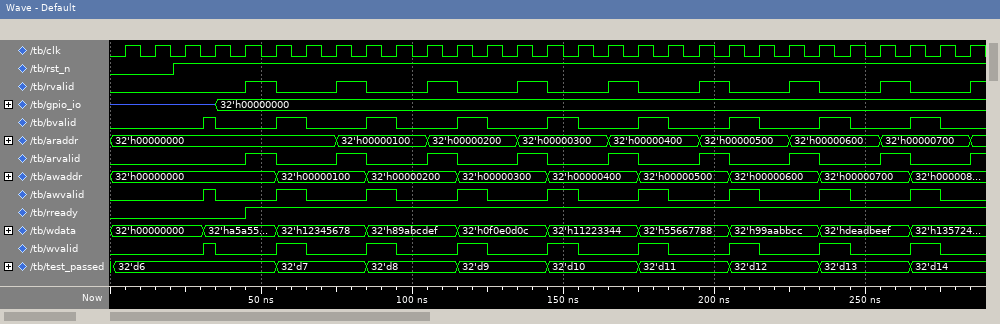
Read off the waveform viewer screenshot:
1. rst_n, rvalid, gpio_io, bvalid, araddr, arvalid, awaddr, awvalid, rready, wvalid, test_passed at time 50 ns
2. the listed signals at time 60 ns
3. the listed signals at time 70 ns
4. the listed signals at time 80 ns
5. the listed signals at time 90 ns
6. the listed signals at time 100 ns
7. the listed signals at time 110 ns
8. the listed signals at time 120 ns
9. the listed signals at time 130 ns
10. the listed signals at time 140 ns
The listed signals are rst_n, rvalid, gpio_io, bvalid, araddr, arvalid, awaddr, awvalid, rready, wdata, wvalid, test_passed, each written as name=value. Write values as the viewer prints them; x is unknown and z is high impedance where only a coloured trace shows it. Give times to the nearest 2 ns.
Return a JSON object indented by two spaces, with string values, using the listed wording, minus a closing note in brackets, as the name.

{
  "rst_n, rvalid, gpio_io, bvalid, araddr, arvalid, awaddr, awvalid, rready, wvalid, test_passed at time 50 ns": "rst_n=1, rvalid=1, gpio_io=32'h00000000, bvalid=0, araddr=32'h00000000, arvalid=1, awaddr=32'h00000000, awvalid=0, rready=1, wvalid=0, test_passed=32'd6",
  "the listed signals at time 60 ns": "rst_n=1, rvalid=0, gpio_io=32'h00000000, bvalid=1, araddr=32'h00000000, arvalid=0, awaddr=32'h00000100, awvalid=1, rready=1, wdata=32'h12345678, wvalid=1, test_passed=32'd7",
  "the listed signals at time 70 ns": "rst_n=1, rvalid=0, gpio_io=32'h00000000, bvalid=0, araddr=32'h00000000, arvalid=0, awaddr=32'h00000100, awvalid=0, rready=1, wdata=32'h12345678, wvalid=0, test_passed=32'd7",
  "the listed signals at time 80 ns": "rst_n=1, rvalid=1, gpio_io=32'h00000000, bvalid=0, araddr=32'h00000100, arvalid=1, awaddr=32'h00000100, awvalid=0, rready=1, wdata=32'h12345678, wvalid=0, test_passed=32'd7",
  "the listed signals at time 90 ns": "rst_n=1, rvalid=0, gpio_io=32'h00000000, bvalid=1, araddr=32'h00000100, arvalid=0, awaddr=32'h00000200, awvalid=1, rready=1, wdata=32'h89abcdef, wvalid=1, test_passed=32'd8",
  "the listed signals at time 100 ns": "rst_n=1, rvalid=0, gpio_io=32'h00000000, bvalid=0, araddr=32'h00000100, arvalid=0, awaddr=32'h00000200, awvalid=0, rready=1, wdata=32'h89abcdef, wvalid=0, test_passed=32'd8",
  "the listed signals at time 110 ns": "rst_n=1, rvalid=1, gpio_io=32'h00000000, bvalid=0, araddr=32'h00000200, arvalid=1, awaddr=32'h00000200, awvalid=0, rready=1, wdata=32'h89abcdef, wvalid=0, test_passed=32'd8",
  "the listed signals at time 120 ns": "rst_n=1, rvalid=0, gpio_io=32'h00000000, bvalid=1, araddr=32'h00000200, arvalid=0, awaddr=32'h00000300, awvalid=1, rready=1, wdata=32'h0f0e0d0c, wvalid=1, test_passed=32'd9",
  "the listed signals at time 130 ns": "rst_n=1, rvalid=0, gpio_io=32'h00000000, bvalid=0, araddr=32'h00000200, arvalid=0, awaddr=32'h00000300, awvalid=0, rready=1, wdata=32'h0f0e0d0c, wvalid=0, test_passed=32'd9",
  "the listed signals at time 140 ns": "rst_n=1, rvalid=1, gpio_io=32'h00000000, bvalid=0, araddr=32'h00000300, arvalid=1, awaddr=32'h00000300, awvalid=0, rready=1, wdata=32'h0f0e0d0c, wvalid=0, test_passed=32'd9"
}
